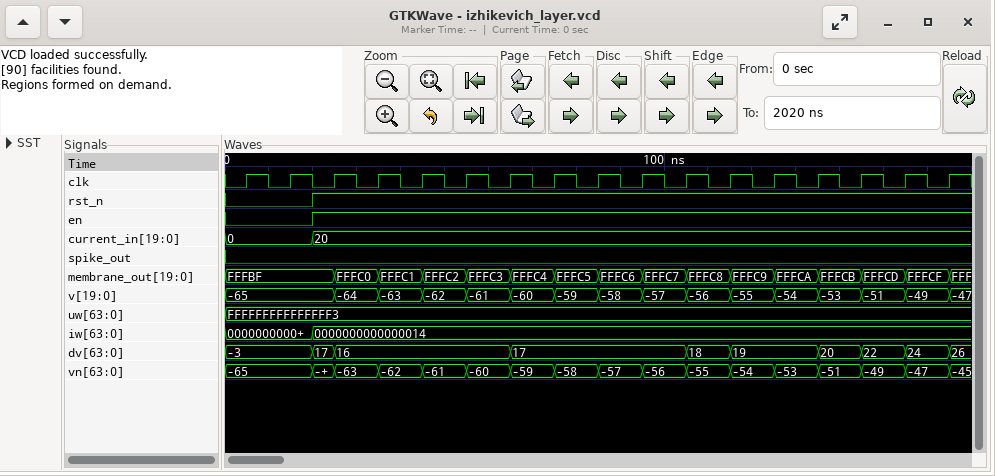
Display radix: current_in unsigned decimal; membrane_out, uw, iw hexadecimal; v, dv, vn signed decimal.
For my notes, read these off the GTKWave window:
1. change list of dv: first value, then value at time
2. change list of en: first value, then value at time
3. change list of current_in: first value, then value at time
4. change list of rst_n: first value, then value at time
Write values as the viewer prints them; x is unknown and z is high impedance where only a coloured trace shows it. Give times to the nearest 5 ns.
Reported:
-3, 17 at 20 ns, 16 at 25 ns, 17 at 65 ns, 18 at 105 ns, 19 at 115 ns, 20 at 135 ns, 22 at 145 ns, 24 at 155 ns, 26 at 165 ns
0, 1 at 20 ns
0, 20 at 20 ns
0, 1 at 20 ns
